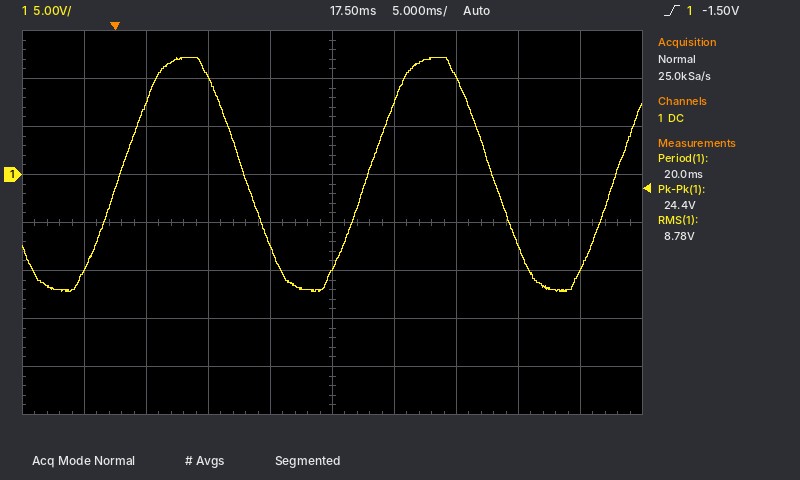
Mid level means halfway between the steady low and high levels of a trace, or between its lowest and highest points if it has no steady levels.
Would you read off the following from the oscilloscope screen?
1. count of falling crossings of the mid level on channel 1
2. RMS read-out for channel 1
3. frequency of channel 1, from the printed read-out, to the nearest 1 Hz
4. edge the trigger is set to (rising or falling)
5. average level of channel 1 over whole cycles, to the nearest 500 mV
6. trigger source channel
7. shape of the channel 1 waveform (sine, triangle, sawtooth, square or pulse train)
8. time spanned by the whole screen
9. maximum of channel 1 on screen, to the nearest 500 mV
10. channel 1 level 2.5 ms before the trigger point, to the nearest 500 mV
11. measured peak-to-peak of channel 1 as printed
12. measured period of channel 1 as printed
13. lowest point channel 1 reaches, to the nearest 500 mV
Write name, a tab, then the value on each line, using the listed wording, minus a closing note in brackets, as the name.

count of falling crossings of the mid level on channel 1	2
RMS read-out for channel 1	8.78 V
frequency of channel 1, from the printed read-out, to the nearest 1 Hz	50 Hz
edge the trigger is set to	rising
average level of channel 1 over whole cycles, to the nearest 500 mV	0.0 V
trigger source channel	channel 1
shape of the channel 1 waveform	sine
time spanned by the whole screen	50 ms
maximum of channel 1 on screen, to the nearest 500 mV	12.0 V
channel 1 level 2.5 ms before the trigger point, to the nearest 500 mV	-10.0 V
measured peak-to-peak of channel 1 as printed	24.4 V
measured period of channel 1 as printed	20.0 ms
lowest point channel 1 reaches, to the nearest 500 mV	-12.0 V
